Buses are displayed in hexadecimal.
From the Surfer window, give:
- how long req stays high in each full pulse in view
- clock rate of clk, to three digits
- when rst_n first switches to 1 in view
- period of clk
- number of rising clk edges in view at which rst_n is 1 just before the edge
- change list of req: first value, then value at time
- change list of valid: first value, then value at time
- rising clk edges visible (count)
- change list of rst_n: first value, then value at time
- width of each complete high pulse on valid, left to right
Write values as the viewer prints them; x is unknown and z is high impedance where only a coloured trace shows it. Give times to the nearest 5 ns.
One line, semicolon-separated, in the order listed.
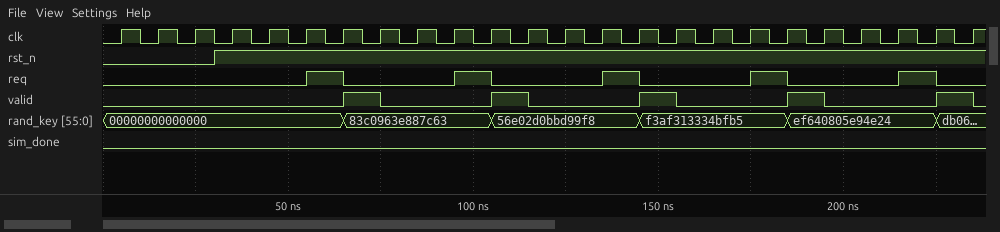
10 ns, 10 ns, 10 ns, 10 ns, 10 ns; 100 MHz; 30 ns; 10 ns; 21; 0, 1 at 55 ns, 0 at 65 ns, 1 at 95 ns, 0 at 105 ns, 1 at 135 ns, 0 at 145 ns, 1 at 175 ns, 0 at 185 ns, 1 at 215 ns, 0 at 225 ns; 0, 1 at 65 ns, 0 at 75 ns, 1 at 105 ns, 0 at 115 ns, 1 at 145 ns, 0 at 155 ns, 1 at 185 ns, 0 at 195 ns, 1 at 225 ns, 0 at 235 ns; 24; 0, 1 at 30 ns; 10 ns, 10 ns, 10 ns, 10 ns, 10 ns
